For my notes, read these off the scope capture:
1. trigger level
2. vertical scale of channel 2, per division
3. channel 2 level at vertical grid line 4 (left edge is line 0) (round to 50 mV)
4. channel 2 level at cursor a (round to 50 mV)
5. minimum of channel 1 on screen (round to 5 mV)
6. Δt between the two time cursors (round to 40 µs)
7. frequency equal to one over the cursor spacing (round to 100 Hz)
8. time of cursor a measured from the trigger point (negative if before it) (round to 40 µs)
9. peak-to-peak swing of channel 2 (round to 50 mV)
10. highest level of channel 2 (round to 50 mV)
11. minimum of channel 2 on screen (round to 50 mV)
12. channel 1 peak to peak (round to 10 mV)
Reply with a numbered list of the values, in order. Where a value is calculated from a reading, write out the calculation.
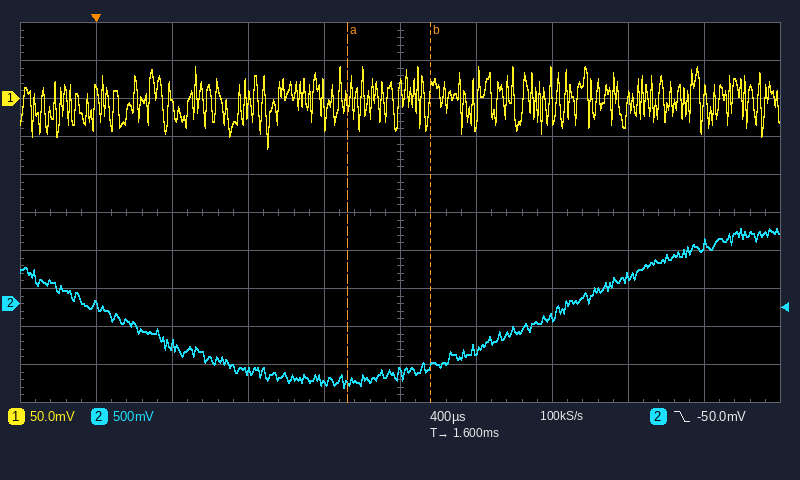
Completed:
1. -50.0 mV
2. 500 mV
3. -1.05 V
4. -1.05 V
5. -65 mV
6. 440 µs
7. 1 / 440 µs ≈ 2.3 kHz
8. +1.32 ms
9. 1.00 V − (-1.10 V) = 2.10 V
10. 1.00 V
11. -1.10 V
12. 110 mV
